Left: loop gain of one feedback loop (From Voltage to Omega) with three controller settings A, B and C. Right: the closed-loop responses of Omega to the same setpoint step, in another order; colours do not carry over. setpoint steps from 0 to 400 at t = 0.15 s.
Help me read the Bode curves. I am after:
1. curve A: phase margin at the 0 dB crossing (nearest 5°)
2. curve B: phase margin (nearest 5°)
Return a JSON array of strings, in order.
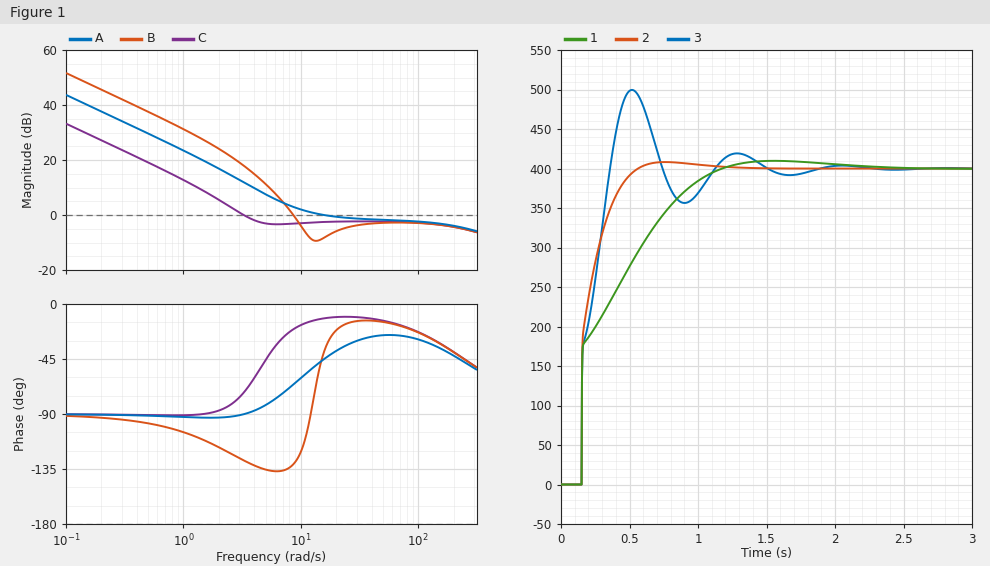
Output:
["135°", "50°"]
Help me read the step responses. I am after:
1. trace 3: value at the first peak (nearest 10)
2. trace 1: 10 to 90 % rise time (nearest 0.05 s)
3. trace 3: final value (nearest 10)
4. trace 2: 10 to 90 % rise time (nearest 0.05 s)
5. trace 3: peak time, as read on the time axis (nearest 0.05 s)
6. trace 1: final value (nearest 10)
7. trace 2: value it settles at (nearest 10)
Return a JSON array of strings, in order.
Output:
["500", "0.70 s", "400", "0.25 s", "0.50 s", "400", "400"]
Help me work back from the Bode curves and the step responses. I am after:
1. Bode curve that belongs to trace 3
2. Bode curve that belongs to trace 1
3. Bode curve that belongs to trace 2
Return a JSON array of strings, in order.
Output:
["B", "C", "A"]
